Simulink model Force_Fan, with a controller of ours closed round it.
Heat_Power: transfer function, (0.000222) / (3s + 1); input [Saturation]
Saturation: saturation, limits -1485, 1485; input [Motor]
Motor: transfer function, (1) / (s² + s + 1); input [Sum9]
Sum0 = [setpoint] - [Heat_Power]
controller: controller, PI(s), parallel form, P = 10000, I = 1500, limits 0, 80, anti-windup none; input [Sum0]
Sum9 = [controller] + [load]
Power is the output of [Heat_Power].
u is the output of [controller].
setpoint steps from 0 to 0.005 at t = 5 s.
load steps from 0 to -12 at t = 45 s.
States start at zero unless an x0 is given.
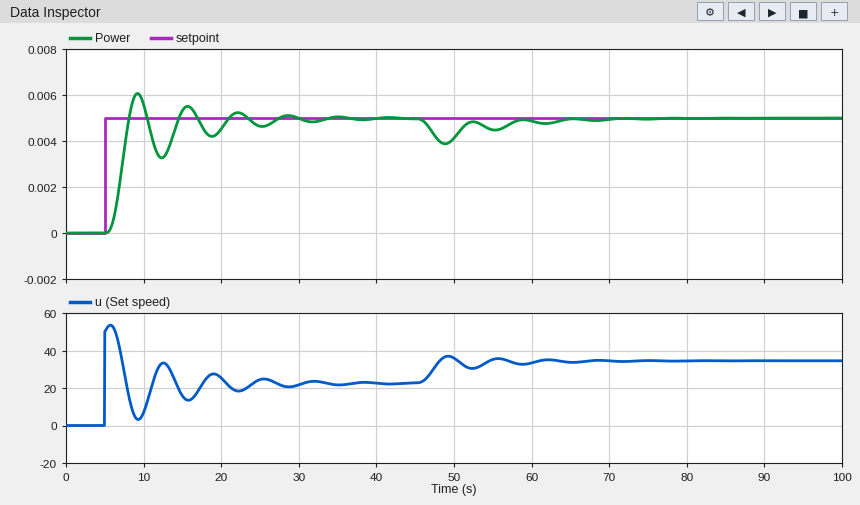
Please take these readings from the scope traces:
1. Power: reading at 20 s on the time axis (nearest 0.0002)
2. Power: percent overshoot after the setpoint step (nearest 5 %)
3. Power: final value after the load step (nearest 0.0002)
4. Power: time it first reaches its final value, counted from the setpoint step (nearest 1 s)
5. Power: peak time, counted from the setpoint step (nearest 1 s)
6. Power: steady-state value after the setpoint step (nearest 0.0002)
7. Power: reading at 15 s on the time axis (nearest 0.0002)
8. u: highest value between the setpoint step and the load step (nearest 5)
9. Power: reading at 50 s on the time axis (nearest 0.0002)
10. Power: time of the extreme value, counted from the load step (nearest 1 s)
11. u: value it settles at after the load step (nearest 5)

0.0046
20 %
0.0050
3 s
4 s
0.0050
0.0054
55
0.0042
4 s
35
